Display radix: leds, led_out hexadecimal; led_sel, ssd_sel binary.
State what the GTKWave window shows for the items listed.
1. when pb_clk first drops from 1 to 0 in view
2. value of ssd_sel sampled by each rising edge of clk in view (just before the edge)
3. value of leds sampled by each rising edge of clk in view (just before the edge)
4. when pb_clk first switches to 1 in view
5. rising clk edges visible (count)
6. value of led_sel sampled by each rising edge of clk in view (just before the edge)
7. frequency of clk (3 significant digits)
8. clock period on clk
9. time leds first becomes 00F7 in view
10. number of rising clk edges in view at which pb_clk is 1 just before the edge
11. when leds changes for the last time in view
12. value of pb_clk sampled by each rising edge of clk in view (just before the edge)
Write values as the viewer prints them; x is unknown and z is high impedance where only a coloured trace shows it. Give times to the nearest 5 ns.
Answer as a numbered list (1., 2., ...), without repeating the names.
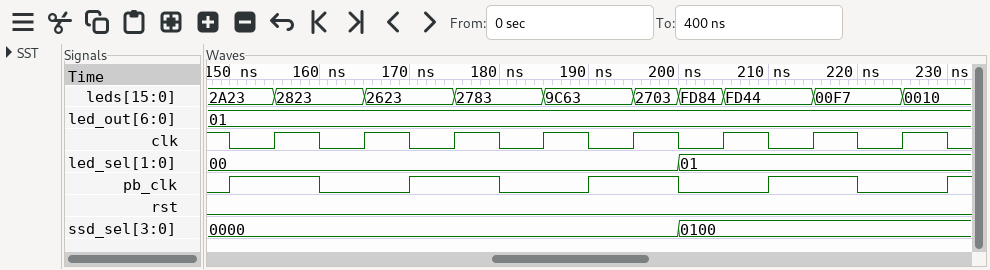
1. 160 ns
2. 0000, 0000, 0000, 0000, 0000, 0100, 0100, 0100
3. 2A23, 2823, 2623, 2783, 9C63, FD84, FD44, 00F7
4. 150 ns
5. 8
6. 00, 00, 00, 00, 00, 01, 01, 01
7. 100 MHz
8. 10 ns
9. 215 ns
10. 4
11. 225 ns
12. 1 0 1 0 1 0 1 0
